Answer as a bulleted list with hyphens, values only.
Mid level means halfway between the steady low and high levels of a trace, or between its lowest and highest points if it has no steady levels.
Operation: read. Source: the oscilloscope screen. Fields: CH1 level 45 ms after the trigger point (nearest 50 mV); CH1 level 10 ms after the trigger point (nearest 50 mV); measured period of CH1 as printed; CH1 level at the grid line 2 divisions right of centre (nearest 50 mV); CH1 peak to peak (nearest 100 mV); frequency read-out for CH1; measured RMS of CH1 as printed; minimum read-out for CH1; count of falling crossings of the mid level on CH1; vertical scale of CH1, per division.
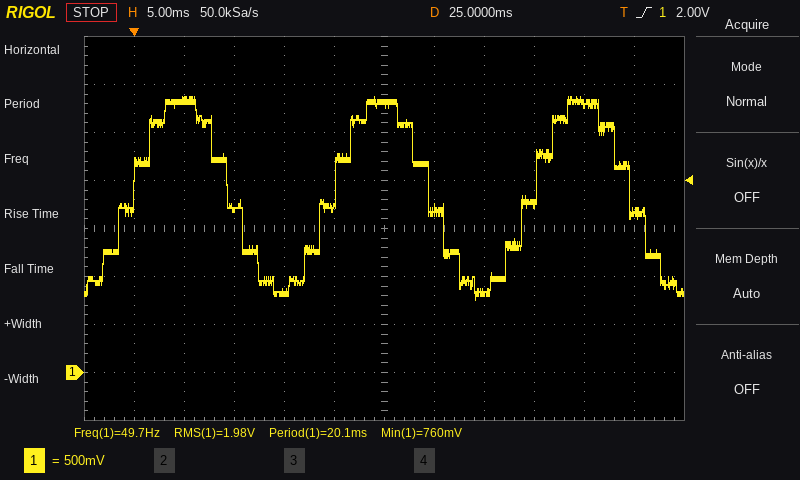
- 2.80 V
- 1.70 V
- 20.1 ms
- 850 mV
- 2.10 V
- 49.7 Hz
- 1.98 V
- 760 mV
- 3
- 500 mV
